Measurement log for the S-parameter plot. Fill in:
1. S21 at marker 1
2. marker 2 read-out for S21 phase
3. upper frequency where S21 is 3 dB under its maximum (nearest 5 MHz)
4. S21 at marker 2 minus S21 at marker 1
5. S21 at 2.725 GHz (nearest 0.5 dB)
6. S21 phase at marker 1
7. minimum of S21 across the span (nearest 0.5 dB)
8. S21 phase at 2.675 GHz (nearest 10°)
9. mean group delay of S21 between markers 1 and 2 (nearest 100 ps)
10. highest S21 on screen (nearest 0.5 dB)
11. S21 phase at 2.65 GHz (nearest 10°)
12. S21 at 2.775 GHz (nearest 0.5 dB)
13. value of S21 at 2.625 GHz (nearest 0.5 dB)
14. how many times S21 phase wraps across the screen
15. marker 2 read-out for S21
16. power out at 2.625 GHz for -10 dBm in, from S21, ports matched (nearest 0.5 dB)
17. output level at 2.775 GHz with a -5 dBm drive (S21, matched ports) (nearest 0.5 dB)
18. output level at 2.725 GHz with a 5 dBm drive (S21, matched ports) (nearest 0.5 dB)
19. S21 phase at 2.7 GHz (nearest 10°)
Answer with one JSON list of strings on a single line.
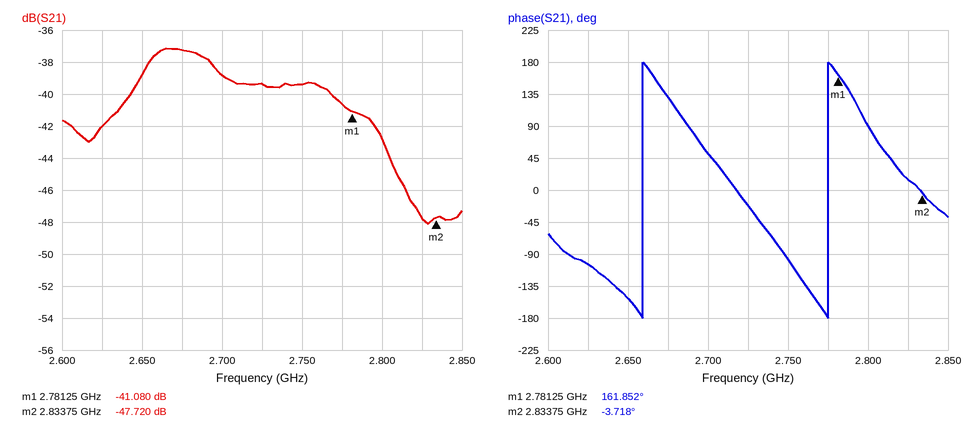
["-41.080 dB", "-3.718°", "2.770 GHz", "-6.640 dB", "-39.5 dB", "161.852°", "-48.0 dB", "130°", "8.8 ns", "-37.0 dB", "-150°", "-40.5 dB", "-42.0 dB", "2", "-47.720 dB", "-52.0 dBm", "-45.5 dBm", "-34.5 dBm", "50°"]
